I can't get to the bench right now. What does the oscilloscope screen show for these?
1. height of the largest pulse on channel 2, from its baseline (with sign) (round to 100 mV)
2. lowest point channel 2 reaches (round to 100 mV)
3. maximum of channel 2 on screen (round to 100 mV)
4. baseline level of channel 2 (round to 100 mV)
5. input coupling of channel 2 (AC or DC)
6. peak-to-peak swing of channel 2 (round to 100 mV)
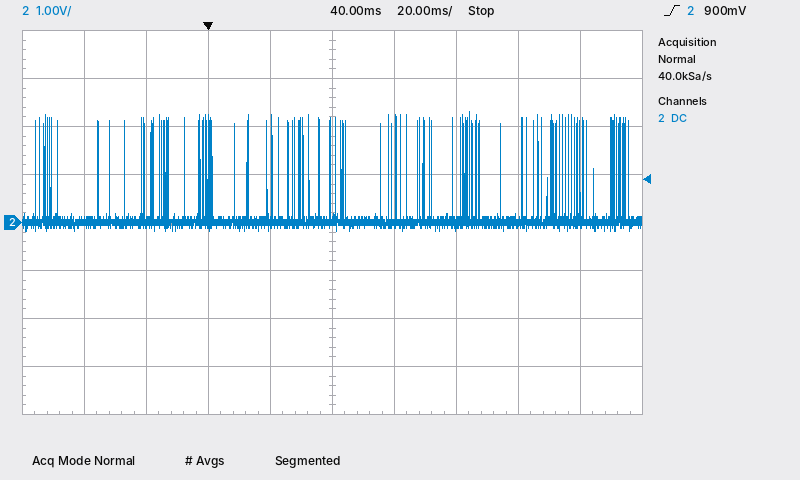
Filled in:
+2.3 V
-200 mV
2.3 V
0.0 V
DC
2.5 V
